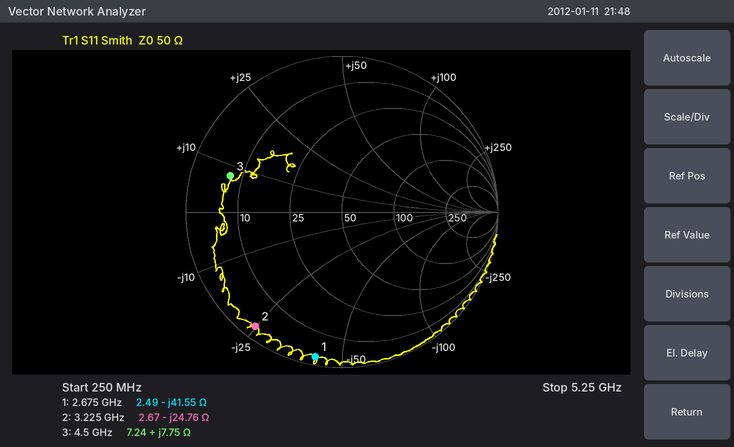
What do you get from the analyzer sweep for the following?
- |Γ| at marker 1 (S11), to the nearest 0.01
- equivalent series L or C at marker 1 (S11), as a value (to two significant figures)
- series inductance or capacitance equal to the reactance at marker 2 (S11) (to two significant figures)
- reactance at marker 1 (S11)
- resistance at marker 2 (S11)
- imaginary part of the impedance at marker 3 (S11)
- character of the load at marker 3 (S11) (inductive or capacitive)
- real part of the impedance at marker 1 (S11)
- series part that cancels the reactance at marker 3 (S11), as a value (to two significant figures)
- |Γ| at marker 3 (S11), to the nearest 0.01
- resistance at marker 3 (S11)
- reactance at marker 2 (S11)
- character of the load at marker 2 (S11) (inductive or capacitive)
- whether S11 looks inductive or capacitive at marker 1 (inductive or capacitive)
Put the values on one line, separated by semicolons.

0.94; 1.4 pF; 2.0 pF; -41.55 Ω; 2.67 Ω; +7.75 Ω; inductive; 2.49 Ω; 4.6 pF; 0.75; 7.24 Ω; -24.76 Ω; capacitive; capacitive
